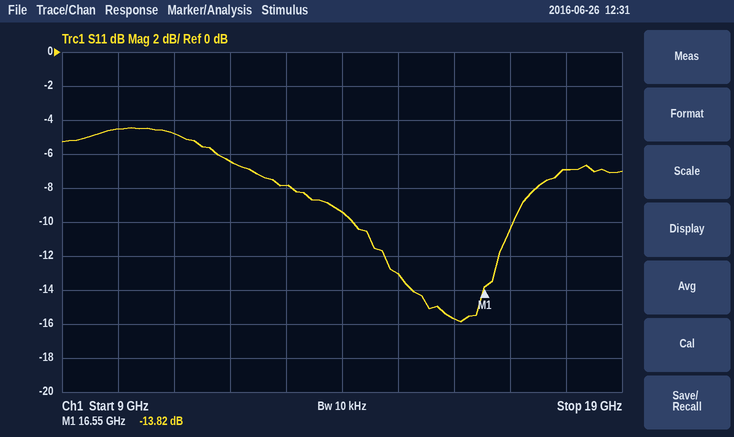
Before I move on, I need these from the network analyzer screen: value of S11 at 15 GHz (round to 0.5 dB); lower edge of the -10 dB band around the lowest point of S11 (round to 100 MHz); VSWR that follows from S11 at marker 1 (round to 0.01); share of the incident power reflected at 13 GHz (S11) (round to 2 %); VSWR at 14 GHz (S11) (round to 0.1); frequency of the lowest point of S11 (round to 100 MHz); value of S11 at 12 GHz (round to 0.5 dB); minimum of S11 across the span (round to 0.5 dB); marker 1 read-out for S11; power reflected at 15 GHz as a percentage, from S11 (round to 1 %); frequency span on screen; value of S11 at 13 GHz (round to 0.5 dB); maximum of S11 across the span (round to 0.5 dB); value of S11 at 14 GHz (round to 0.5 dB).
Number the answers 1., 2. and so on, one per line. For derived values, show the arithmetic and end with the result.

1. -13.0 dB
2. 14.2 GHz
3. (1 + 0.2037)/(1 − 0.2037) ≈ 1.51
4. 10^(-8/10) ≈ 16 %
5. |Γ| = 10^(-9.5/20) = 0.3350; VSWR = (1 + 0.3350)/(1 − 0.3350) ≈ 2.0
6. 16.1 GHz
7. -6.5 dB
8. -16.0 dB
9. -13.82 dB
10. 10^(-13/10) ≈ 5 %
11. 10 GHz
12. -8.0 dB
13. -4.5 dB
14. -9.5 dB
